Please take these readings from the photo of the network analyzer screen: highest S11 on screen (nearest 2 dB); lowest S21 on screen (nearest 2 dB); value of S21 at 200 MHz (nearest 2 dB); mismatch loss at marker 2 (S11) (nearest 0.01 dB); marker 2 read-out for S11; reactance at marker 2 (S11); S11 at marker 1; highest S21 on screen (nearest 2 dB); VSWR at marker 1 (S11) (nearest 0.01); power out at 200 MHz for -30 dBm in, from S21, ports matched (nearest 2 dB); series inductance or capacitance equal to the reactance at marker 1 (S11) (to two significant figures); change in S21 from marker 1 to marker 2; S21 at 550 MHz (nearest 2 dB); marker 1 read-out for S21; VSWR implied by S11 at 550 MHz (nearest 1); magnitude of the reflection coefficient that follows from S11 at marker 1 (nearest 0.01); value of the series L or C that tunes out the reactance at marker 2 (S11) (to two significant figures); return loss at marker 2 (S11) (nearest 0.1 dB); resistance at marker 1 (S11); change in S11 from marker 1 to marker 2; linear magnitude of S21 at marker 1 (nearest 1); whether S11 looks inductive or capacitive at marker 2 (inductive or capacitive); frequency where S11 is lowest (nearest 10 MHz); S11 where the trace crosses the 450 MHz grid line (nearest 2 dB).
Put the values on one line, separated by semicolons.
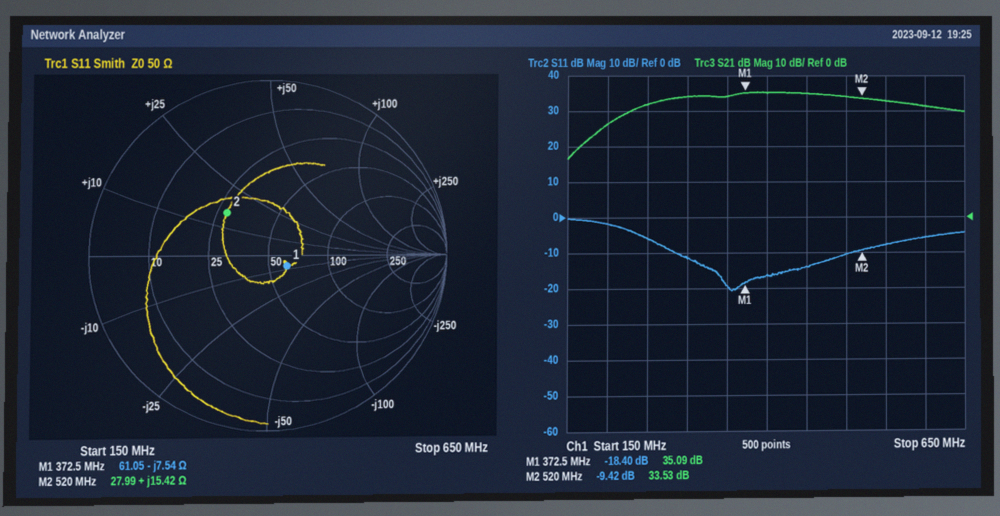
0 dB; 16 dB; 26 dB; 0.53 dB; -9.42 dB; +15.42 Ω; -18.40 dB; 36 dB; 1.27; -4 dBm; 57 pF; -1.56 dB; 32 dB; 35.09 dB; 2; 0.12; 20 pF; 9.4 dB; 61.05 Ω; 8.98 dB; 57; inductive; 360 MHz; -14 dB
